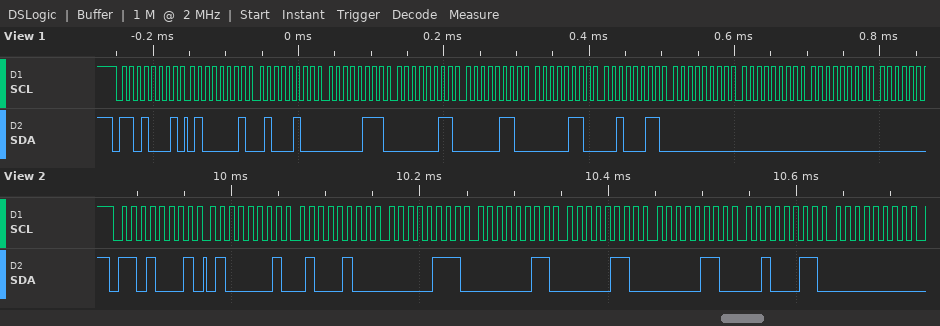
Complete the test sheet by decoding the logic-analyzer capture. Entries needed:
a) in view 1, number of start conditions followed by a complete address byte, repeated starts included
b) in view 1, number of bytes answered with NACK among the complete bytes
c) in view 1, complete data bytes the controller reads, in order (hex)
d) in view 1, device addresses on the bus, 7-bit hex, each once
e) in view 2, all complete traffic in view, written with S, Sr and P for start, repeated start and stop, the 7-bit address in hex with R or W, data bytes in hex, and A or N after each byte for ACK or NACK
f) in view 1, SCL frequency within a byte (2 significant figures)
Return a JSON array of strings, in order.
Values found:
["1", "0", "41 44 07 03 06 06 23 00 00 00", "0x68", "S 68R A 41 A 44 A 07 A 03 A 06 A 06 A 23 A 00 A", "100 kHz"]
